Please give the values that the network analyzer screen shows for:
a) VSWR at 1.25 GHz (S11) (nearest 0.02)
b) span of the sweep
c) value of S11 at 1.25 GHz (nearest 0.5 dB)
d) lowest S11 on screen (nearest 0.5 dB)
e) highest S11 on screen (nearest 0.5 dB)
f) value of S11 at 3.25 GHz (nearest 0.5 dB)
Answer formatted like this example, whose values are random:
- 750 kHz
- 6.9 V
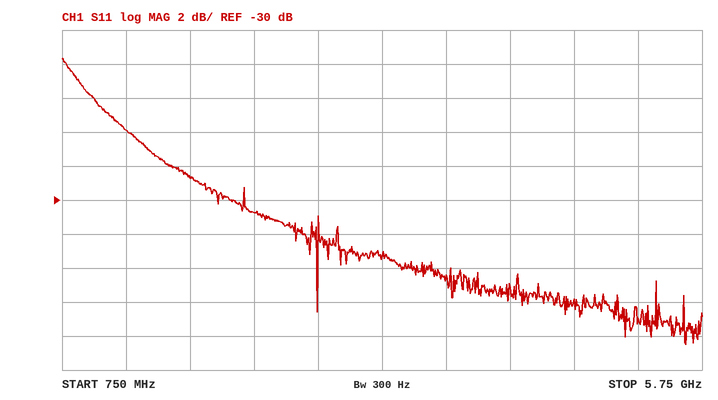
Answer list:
- 1.10
- 5 GHz
- -26.0 dB
- -38.5 dB
- -21.5 dB
- -33.5 dB
